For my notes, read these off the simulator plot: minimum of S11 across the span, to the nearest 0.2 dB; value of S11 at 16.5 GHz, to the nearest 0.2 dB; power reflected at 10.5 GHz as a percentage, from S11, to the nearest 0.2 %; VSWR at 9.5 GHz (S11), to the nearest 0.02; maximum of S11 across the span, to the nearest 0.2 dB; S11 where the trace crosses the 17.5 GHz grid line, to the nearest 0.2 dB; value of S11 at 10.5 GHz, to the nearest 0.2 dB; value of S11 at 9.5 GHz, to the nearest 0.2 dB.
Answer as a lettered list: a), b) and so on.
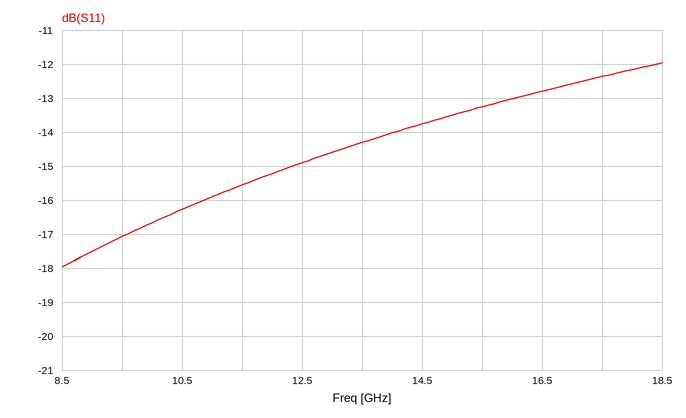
a) -18.0 dB
b) -12.8 dB
c) 2.4 %
d) 1.32
e) -12.0 dB
f) -12.4 dB
g) -16.2 dB
h) -17.0 dB
